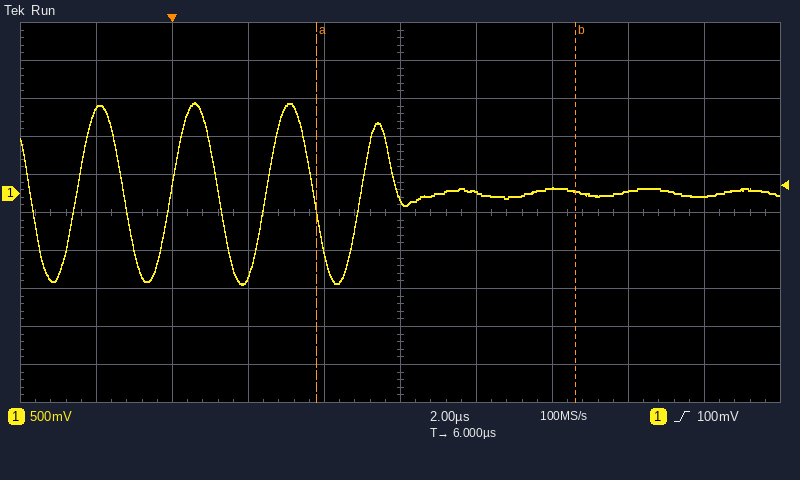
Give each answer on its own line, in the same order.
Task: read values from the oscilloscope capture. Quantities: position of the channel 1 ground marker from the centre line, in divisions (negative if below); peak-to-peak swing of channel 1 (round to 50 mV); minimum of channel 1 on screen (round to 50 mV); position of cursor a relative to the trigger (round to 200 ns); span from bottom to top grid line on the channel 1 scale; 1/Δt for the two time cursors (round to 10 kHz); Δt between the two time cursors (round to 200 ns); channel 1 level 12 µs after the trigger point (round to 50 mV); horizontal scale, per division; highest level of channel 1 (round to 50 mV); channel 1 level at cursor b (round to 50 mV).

+0.5 div
2.40 V
-1.20 V
+3.8 µs
5 V
150 kHz
6.8 µs
50 mV
2 µs
1.20 V
50 mV
